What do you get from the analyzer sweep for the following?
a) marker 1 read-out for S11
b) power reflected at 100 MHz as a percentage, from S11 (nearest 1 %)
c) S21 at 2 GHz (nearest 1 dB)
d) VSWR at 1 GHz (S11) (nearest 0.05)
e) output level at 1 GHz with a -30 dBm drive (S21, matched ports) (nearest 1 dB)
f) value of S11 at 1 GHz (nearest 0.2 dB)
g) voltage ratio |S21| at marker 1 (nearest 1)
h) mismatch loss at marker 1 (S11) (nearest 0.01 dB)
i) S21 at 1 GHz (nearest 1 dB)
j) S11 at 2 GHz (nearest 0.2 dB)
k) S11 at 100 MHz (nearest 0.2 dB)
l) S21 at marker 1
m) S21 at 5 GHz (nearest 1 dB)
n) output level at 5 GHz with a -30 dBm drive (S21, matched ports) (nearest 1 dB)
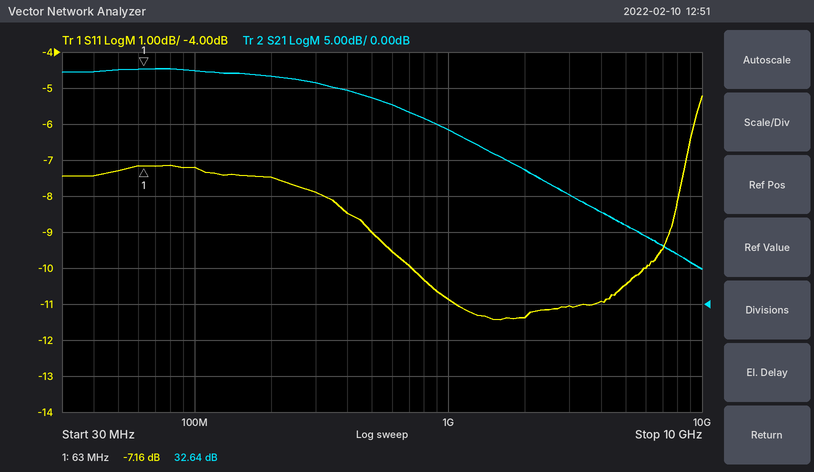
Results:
-7.16 dB
19 %
19 dB
1.80
-6 dBm
-10.8 dB
43
0.93 dB
24 dB
-11.4 dB
-7.2 dB
32.64 dB
11 dB
-19 dBm
